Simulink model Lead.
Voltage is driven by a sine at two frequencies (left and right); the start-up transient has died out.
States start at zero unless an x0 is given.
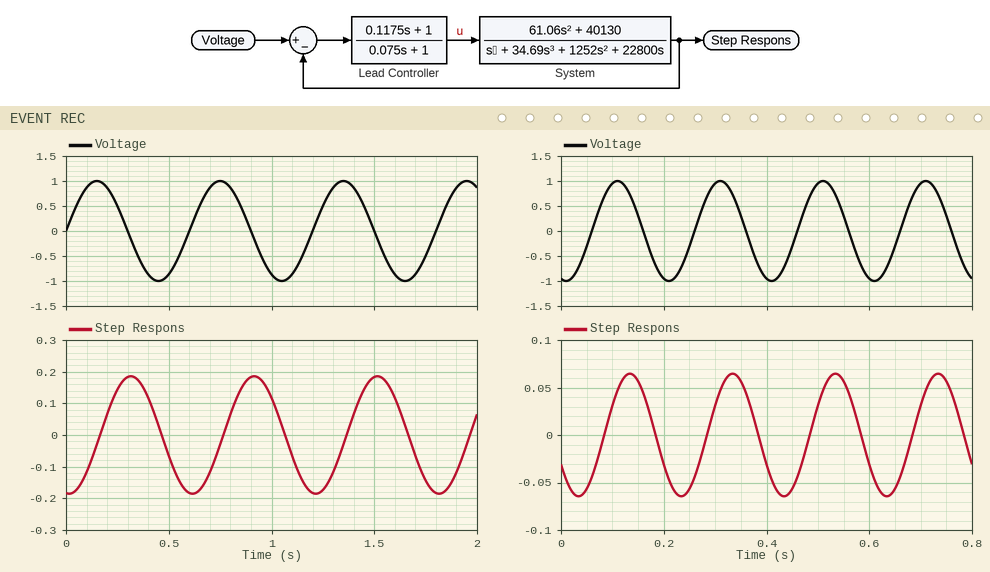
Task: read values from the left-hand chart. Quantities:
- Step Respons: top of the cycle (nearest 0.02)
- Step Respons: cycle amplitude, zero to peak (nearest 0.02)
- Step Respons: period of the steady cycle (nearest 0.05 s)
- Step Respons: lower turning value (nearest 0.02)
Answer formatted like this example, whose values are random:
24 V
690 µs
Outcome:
0.18
0.18
0.60 s
-0.18
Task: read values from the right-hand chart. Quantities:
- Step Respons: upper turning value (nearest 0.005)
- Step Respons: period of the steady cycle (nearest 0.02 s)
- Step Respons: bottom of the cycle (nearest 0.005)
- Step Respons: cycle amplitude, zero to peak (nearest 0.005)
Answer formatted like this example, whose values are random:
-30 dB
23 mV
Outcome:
0.065
0.20 s
-0.065
0.065
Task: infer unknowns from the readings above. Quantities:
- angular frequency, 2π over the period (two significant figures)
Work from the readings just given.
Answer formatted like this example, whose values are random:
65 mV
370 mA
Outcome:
31 rad/s
